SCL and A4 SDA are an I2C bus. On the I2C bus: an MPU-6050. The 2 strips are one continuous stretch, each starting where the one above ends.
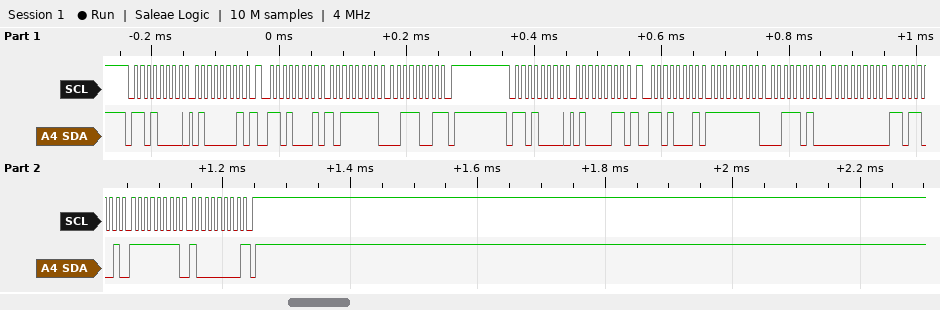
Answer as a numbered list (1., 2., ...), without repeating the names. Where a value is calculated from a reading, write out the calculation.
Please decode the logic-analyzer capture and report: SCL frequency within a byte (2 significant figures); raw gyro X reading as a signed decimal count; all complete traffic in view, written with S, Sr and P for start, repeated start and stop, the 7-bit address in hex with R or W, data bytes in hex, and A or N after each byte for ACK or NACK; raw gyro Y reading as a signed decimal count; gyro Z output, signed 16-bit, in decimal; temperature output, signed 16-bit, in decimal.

1. 100 kHz
2. 0xFF3A = -198
3. S 68W A 41 A Sr 68R A BF A 39 N P S 68W A 43 A Sr 68R A FF A 3A A 00 A D9 A FF A 80 N P
4. 0x00D9 = 217
5. 0xFF80 = -128
6. 0xBF39 = -16583
